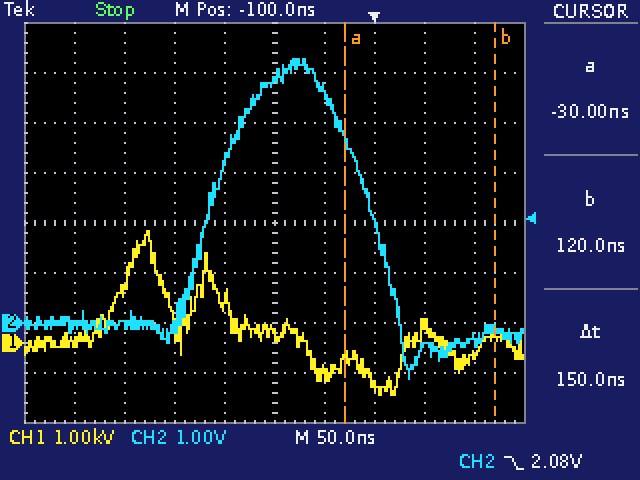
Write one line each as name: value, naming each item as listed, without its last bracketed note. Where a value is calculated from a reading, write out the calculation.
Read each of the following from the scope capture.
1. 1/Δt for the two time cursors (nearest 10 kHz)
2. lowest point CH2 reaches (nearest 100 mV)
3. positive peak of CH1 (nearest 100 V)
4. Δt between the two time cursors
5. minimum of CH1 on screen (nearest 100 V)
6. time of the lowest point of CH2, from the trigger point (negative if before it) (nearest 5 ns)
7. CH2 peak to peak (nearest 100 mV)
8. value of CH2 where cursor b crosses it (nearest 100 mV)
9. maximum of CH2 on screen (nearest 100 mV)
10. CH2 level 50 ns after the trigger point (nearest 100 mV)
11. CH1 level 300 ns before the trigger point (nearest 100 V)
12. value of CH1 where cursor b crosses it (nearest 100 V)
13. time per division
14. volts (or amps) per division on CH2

1/Δt for the two time cursors: 1 / 150 ns ≈ 6.67 MHz
lowest point CH2 reaches: -1.1 V
positive peak of CH1: 2.2 kV
Δt between the two time cursors: 150 ns
minimum of CH1 on screen: -1.0 kV
time of the lowest point of CH2, from the trigger point (negative if before it): +35 ns
CH2 peak to peak: 5.3 V − (-1.1 V) = 6.4 V
value of CH2 where cursor b crosses it: -100 mV
maximum of CH2 on screen: 5.3 V
CH2 level 50 ns after the trigger point: -500 mV
CH1 level 300 ns before the trigger point: 0.0 kV
value of CH1 where cursor b crosses it: 100 V
time per division: 50 ns
volts (or amps) per division on CH2: 1 V
